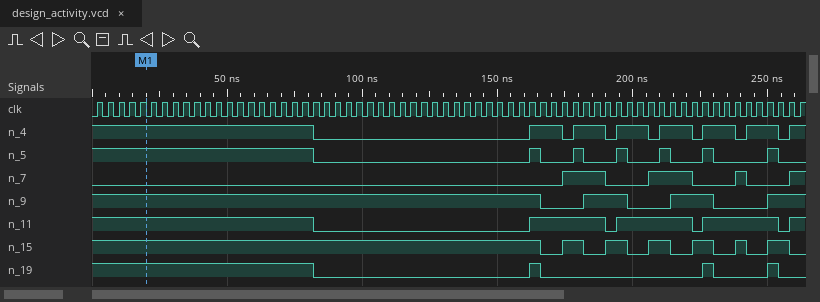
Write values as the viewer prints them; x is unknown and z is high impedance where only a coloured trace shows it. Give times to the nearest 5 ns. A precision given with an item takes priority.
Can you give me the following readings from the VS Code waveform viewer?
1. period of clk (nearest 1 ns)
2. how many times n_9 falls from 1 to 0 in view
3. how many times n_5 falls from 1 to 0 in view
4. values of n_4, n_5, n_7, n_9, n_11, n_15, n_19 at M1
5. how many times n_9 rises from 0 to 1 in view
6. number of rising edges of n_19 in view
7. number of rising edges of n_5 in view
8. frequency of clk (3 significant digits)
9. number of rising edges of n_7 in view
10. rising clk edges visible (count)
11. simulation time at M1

4 ns
3
7
n_4=1, n_5=1, n_7=0, n_9=1, n_11=1, n_15=1, n_19=1
3
3
6
250 MHz
4
66
20 ns
